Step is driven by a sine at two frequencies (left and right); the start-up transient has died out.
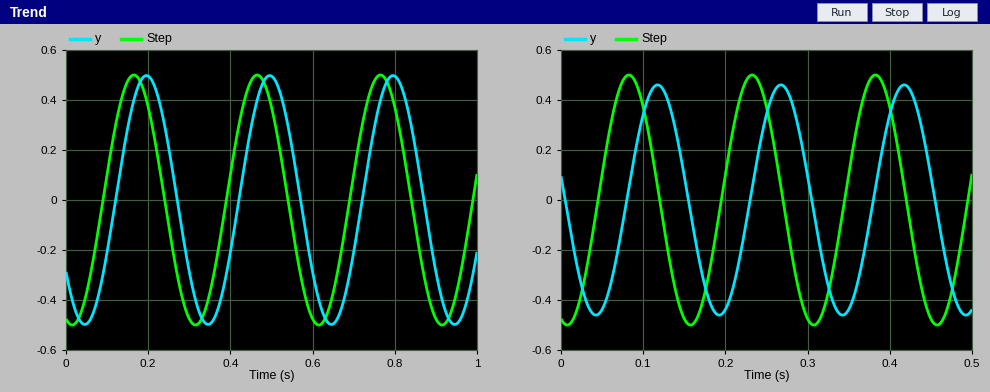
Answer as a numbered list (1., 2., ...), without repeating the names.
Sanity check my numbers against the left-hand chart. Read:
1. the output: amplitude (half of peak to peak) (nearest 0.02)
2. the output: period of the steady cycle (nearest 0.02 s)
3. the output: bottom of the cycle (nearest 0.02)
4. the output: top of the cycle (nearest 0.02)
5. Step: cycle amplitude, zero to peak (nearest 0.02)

1. 0.50
2. 0.30 s
3. -0.50
4. 0.50
5. 0.50
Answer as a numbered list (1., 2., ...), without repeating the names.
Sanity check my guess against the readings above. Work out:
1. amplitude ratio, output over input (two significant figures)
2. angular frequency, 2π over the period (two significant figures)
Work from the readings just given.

1. 1.0
2. 21 rad/s
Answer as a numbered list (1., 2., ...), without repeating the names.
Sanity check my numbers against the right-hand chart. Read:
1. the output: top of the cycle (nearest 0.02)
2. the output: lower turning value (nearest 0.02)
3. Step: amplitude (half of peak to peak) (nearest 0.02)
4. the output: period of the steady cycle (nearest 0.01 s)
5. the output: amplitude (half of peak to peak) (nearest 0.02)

1. 0.46
2. -0.46
3. 0.50
4. 0.15 s
5. 0.46
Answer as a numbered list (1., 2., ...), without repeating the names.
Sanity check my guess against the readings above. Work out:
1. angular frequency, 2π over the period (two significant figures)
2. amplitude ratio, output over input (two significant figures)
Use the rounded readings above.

1. 42 rad/s
2. 0.92
